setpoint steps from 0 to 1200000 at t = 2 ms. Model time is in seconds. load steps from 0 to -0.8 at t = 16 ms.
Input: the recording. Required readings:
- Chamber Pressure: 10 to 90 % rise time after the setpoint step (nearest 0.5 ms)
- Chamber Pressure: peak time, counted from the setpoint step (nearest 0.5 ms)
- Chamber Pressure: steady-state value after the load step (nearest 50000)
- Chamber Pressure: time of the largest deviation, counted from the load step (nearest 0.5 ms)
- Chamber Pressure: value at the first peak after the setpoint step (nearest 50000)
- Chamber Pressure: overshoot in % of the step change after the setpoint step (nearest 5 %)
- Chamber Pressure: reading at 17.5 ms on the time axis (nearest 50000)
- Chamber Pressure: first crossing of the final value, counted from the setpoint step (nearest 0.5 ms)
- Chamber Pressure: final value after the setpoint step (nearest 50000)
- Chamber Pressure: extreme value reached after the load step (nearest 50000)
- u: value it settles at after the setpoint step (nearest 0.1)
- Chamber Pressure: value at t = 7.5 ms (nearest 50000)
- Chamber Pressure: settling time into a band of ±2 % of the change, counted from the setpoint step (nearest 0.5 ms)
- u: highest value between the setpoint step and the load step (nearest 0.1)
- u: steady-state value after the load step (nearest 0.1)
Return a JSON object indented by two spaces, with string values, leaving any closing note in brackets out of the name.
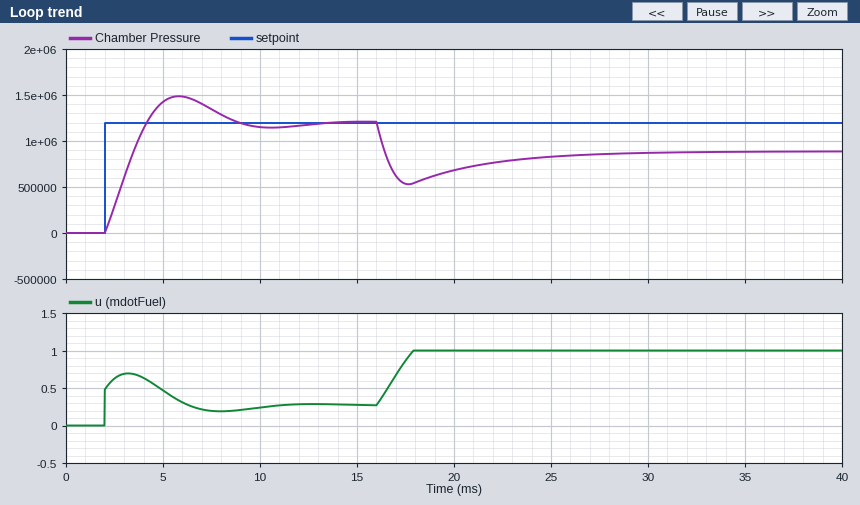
{
  "Chamber Pressure: 10 to 90 % rise time after the setpoint step": "1.5 ms",
  "Chamber Pressure: peak time, counted from the setpoint step": "4.0 ms",
  "Chamber Pressure: steady-state value after the load step": "900000",
  "Chamber Pressure: time of the largest deviation, counted from the load step": "1.5 ms",
  "Chamber Pressure: value at the first peak after the setpoint step": "1500000",
  "Chamber Pressure: overshoot in % of the step change after the setpoint step": "25 %",
  "Chamber Pressure: reading at 17.5 ms on the time axis": "550000",
  "Chamber Pressure: first crossing of the final value, counted from the setpoint step": "2.0 ms",
  "Chamber Pressure: final value after the setpoint step": "1200000",
  "Chamber Pressure: extreme value reached after the load step": "550000",
  "u: value it settles at after the setpoint step": "0.3",
  "Chamber Pressure: value at t = 7.5 ms": "1350000",
  "Chamber Pressure: settling time into a band of ±2 % of the change, counted from the setpoint step": "10.5 ms",
  "u: highest value between the setpoint step and the load step": "0.7",
  "u: steady-state value after the load step": "1.0"
}
